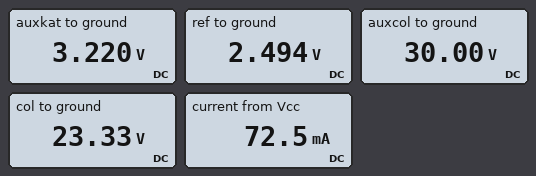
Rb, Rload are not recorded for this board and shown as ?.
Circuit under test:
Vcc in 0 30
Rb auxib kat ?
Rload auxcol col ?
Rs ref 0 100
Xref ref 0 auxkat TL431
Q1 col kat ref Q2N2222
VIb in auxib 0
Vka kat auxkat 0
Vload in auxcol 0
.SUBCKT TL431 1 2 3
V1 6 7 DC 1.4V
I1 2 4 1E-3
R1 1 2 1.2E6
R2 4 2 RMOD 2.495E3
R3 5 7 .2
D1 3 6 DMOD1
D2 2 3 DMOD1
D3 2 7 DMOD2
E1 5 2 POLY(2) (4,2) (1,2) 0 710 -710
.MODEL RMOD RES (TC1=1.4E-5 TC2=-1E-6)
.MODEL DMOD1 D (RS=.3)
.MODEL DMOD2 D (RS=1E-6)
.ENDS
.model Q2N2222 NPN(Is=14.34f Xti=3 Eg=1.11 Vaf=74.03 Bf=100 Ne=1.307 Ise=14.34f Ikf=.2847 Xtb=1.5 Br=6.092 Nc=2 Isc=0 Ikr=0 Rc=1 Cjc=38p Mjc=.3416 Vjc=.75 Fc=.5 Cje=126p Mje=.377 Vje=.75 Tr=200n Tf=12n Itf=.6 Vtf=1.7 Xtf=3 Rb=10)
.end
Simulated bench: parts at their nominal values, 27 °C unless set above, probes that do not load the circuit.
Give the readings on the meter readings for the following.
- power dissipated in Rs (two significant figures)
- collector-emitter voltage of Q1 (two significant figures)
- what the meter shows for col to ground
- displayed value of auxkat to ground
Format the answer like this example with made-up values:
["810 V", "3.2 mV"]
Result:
["62 mW", "21 V", "23.33 V", "3.220 V"]
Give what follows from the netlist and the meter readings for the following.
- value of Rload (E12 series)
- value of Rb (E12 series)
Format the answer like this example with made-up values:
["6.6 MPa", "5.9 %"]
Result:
["270 Ω", "560 Ω"]
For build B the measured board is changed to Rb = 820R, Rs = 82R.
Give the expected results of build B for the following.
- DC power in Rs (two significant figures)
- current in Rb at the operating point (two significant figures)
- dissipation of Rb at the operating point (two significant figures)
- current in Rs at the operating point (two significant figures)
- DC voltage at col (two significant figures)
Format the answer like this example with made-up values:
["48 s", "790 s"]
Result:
["76 mW", "33 mA", "870 mW", "30 mA", "22 V"]
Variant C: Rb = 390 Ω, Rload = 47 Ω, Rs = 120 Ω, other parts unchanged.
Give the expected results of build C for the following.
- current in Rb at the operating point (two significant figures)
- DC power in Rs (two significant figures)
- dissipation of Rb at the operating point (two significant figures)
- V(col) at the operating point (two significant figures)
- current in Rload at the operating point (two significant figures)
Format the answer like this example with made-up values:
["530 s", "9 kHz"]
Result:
["69 mA", "52 mW", "1.8 W", "29 V", "21 mA"]
